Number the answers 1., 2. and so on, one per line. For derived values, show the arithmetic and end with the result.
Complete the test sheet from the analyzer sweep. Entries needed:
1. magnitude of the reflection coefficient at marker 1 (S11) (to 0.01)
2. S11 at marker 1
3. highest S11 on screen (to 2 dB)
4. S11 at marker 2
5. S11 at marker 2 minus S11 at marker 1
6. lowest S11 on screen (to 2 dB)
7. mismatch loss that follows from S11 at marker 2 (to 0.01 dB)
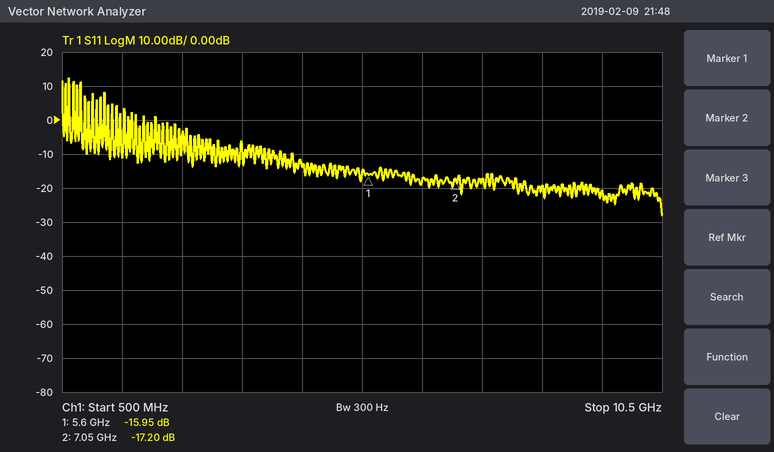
1. 10^(-15.95/20) ≈ 0.16
2. -15.95 dB
3. 12 dB
4. -17.20 dB
5. -17.2 − (-15.95) = -1.25 dB
6. -28 dB
7. −10 log10(1 − 10^(-17.2/10)) ≈ 0.08 dB
